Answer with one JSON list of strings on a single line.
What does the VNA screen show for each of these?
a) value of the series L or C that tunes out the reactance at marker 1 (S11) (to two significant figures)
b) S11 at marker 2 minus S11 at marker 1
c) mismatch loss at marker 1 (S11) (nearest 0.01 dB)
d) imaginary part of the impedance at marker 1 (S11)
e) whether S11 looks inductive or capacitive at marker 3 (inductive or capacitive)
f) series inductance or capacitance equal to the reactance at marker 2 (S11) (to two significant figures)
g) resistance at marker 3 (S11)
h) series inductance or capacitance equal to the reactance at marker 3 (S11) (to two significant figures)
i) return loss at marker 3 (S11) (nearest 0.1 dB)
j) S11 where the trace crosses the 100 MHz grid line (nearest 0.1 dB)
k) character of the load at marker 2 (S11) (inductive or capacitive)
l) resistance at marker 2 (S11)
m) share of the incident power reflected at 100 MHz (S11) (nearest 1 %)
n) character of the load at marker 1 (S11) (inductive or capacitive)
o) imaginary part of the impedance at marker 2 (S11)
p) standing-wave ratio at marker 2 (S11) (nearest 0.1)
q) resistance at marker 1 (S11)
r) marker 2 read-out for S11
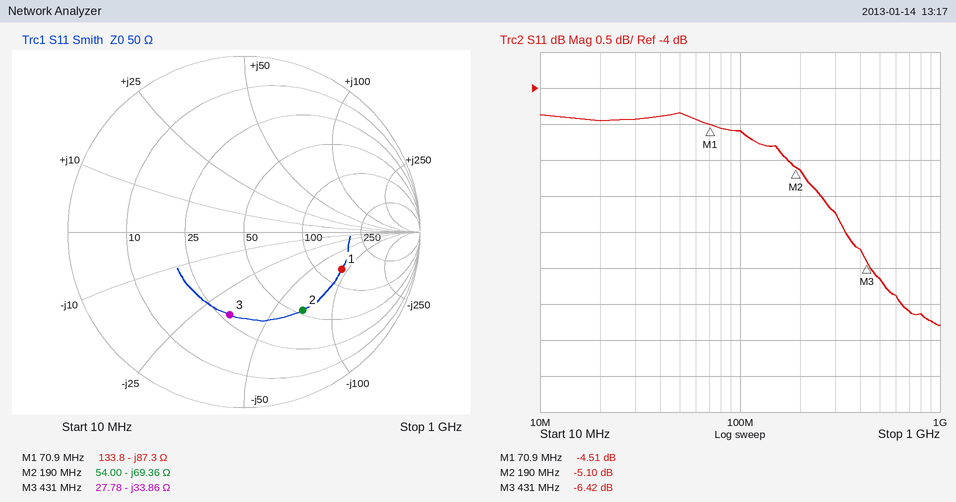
["200 nH", "-0.59 dB", "1.90 dB", "-87.3 Ω", "capacitive", "12 pF", "27.78 Ω", "11 pF", "6.4 dB", "-4.6 dB", "capacitive", "54.00 Ω", "35 %", "capacitive", "-69.36 Ω", "3.5", "133.8 Ω", "-5.10 dB"]
